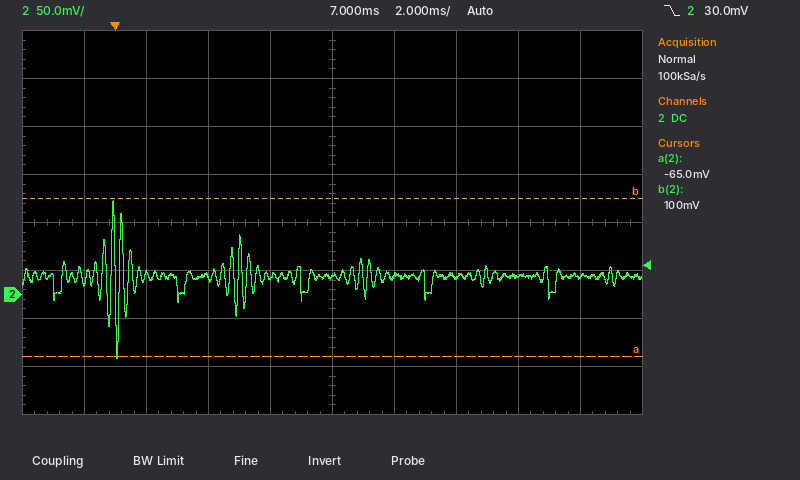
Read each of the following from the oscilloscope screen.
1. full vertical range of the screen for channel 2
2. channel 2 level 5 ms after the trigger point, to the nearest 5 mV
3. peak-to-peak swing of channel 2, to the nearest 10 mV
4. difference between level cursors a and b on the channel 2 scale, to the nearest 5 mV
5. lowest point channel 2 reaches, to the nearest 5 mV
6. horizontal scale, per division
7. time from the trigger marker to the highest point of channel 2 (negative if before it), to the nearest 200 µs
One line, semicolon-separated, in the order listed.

400 mV; 20 mV; 160 mV; 165 mV; -65 mV; 2 ms; 0.0 ms
